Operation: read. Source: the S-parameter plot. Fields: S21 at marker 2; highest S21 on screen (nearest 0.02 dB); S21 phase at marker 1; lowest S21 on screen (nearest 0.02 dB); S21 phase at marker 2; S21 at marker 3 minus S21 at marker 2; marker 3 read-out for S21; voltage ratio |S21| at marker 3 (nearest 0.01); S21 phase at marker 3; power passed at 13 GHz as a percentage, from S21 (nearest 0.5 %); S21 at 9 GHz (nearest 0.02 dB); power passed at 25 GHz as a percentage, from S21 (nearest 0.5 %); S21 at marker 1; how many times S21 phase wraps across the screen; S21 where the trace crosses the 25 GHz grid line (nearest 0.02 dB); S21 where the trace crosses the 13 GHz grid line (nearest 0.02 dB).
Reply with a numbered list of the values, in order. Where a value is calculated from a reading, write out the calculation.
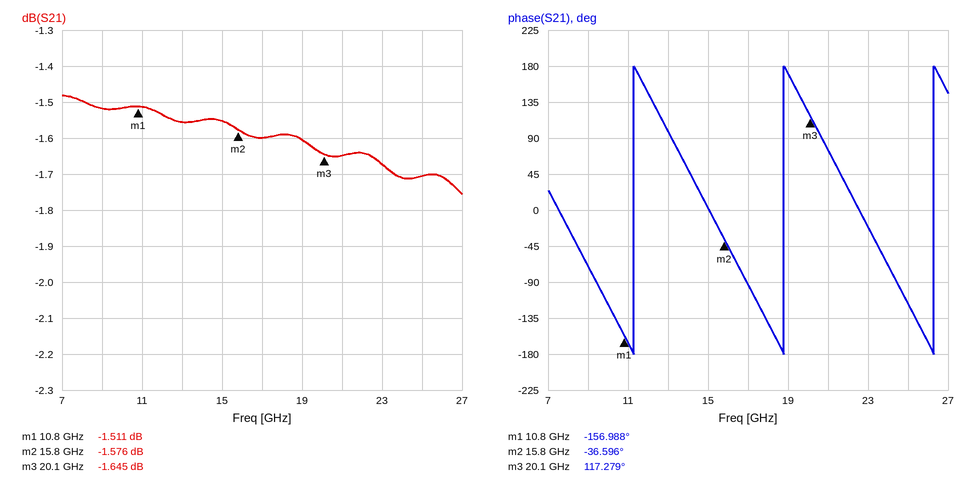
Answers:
1. -1.576 dB
2. -1.48 dB
3. -156.988°
4. -1.76 dB
5. -36.596°
6. -1.645 − (-1.576) = -0.069 dB
7. -1.645 dB
8. 10^(-1.645/20) ≈ 0.83
9. 117.279°
10. 10^(-1.56/10) ≈ 69.8 %, so 70.0 % to the nearest 0.5 %
11. -1.52 dB
12. 10^(-1.7/10) ≈ 67.6 %, so 67.5 % to the nearest 0.5 %
13. -1.511 dB
14. 3
15. -1.70 dB
16. -1.56 dB
